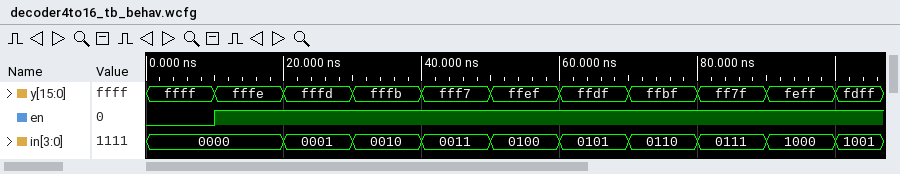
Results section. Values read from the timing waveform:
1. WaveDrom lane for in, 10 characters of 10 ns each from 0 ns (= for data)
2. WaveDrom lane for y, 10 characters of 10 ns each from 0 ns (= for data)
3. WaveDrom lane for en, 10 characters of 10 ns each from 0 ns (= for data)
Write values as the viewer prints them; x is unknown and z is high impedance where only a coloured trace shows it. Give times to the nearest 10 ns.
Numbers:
{name: 'in', wave: '=.========', data: '0000 0001 0010 0011 0100 0101 0110 0111 1000'}
{name: 'y', wave: '==========', data: 'ffff fffe fffd fffb fff7 ffef ffdf ffbf ff7f feff'}
{name: 'en', wave: '01........'}
